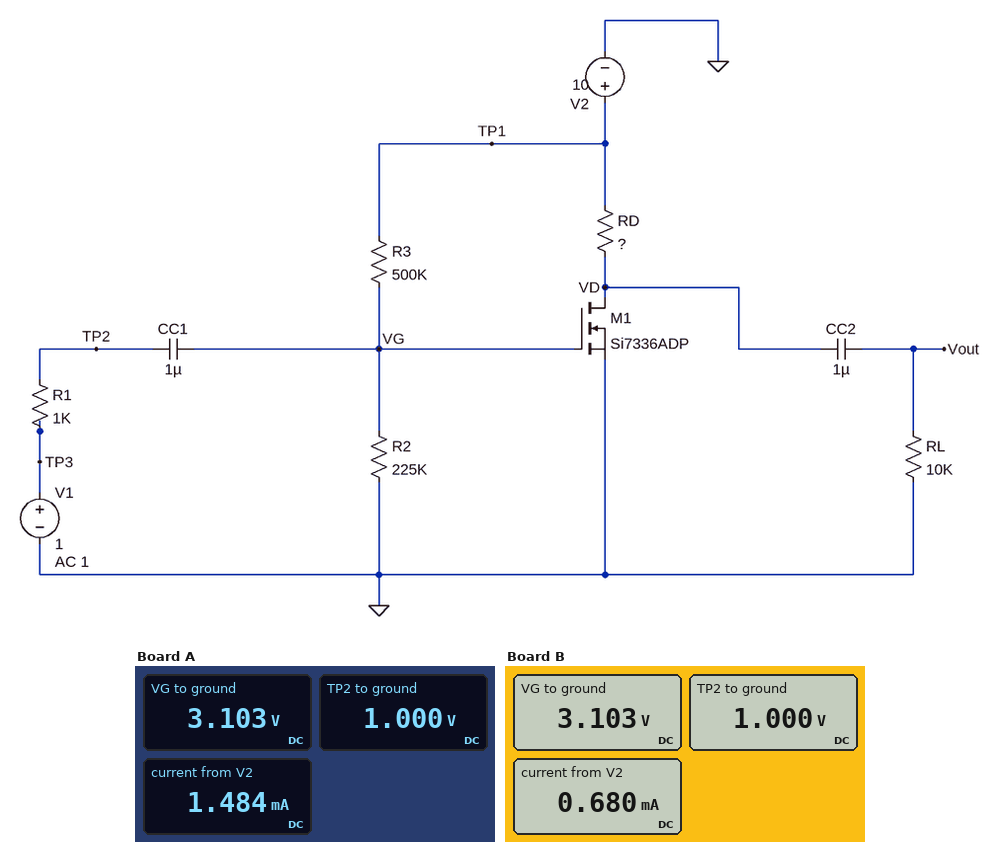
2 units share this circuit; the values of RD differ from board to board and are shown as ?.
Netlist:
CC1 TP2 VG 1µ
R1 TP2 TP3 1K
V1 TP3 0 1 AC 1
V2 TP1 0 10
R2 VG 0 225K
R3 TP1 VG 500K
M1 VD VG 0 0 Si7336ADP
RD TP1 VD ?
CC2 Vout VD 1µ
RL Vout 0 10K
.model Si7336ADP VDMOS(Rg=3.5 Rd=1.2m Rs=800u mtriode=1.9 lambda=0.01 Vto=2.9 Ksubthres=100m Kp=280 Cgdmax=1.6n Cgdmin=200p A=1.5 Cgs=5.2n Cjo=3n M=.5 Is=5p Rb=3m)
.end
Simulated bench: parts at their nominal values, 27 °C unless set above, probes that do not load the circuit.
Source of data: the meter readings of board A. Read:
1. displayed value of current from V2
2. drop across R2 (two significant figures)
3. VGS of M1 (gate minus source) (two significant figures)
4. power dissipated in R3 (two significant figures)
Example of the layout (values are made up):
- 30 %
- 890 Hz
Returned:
- 1.484 mA
- 3.1 V
- 3.1 V
- 95 µW
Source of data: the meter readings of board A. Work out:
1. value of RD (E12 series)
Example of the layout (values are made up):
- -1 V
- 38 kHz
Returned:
- 6.8 kΩ
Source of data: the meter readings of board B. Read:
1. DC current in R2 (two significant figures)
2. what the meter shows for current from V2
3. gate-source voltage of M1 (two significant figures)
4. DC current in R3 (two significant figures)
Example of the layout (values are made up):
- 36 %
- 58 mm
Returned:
- 14 µA
- 0.680 mA
- 3.1 V
- 14 µA
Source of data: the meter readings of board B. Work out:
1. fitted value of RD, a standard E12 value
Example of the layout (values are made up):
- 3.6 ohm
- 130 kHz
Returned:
- 15 kΩ
